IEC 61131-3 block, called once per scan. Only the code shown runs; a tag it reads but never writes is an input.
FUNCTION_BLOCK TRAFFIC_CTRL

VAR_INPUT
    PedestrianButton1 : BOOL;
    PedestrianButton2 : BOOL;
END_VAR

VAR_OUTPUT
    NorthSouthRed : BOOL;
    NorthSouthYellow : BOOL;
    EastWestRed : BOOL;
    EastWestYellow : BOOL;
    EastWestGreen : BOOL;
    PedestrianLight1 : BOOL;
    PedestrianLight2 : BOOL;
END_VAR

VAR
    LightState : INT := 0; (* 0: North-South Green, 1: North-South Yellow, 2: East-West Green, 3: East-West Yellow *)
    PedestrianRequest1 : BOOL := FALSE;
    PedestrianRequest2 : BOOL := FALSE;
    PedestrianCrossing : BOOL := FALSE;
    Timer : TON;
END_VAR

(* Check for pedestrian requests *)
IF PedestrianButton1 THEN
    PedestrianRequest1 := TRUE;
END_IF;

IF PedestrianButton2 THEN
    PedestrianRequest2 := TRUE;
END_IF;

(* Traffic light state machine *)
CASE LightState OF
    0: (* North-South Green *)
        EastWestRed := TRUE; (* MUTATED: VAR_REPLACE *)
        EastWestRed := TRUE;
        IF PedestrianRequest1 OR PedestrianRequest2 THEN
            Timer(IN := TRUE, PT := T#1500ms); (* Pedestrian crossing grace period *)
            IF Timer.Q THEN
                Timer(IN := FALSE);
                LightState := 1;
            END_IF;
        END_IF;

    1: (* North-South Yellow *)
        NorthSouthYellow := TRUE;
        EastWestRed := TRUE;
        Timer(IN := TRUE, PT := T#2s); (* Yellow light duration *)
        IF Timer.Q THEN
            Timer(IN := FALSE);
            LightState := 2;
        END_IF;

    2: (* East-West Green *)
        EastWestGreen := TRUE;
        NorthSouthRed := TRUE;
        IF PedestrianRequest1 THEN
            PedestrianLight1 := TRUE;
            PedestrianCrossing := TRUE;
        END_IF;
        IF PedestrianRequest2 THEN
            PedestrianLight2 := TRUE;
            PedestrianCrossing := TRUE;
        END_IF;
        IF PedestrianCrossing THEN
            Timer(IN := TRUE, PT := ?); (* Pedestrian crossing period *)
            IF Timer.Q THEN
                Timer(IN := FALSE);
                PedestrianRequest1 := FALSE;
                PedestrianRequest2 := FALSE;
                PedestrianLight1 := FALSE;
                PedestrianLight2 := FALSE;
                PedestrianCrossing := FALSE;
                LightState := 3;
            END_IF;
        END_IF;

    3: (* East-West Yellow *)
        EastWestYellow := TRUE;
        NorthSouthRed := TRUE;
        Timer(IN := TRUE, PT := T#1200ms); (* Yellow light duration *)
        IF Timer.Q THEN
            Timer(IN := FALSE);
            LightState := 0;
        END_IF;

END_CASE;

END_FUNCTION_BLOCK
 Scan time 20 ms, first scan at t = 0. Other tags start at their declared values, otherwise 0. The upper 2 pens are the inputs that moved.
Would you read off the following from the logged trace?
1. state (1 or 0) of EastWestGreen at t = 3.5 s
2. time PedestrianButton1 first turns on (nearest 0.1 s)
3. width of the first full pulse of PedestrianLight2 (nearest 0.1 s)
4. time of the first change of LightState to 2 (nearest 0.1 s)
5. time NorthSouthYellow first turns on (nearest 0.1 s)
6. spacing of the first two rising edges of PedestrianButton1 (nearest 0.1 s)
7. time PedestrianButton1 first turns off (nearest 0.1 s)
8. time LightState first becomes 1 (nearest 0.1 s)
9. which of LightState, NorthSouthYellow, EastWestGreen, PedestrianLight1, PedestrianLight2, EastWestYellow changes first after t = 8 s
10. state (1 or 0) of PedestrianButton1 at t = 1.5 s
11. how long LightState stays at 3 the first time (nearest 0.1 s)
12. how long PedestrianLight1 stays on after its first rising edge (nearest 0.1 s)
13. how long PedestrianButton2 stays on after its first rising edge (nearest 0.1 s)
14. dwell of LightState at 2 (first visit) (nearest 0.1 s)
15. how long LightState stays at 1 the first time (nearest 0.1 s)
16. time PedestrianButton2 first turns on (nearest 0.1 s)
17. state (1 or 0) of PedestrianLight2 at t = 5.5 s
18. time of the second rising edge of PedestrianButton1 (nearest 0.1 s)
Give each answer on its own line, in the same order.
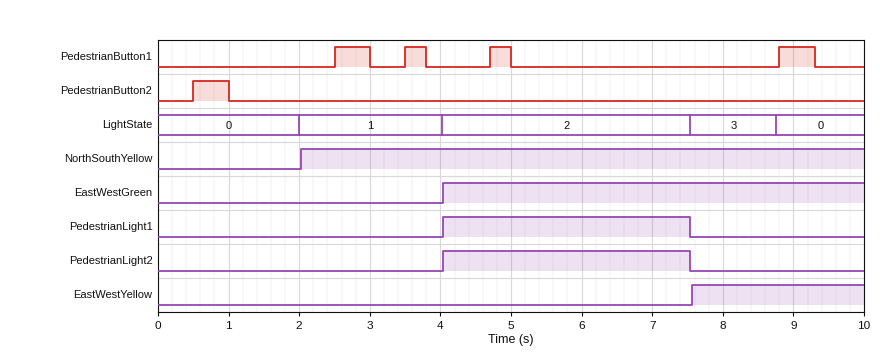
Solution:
0
2.5 s
3.5 s
4.0 s
2.0 s
1.0 s
3.0 s
2.0 s
LightState
0
1.2 s
3.5 s
0.5 s
3.5 s
2.0 s
0.5 s
1
3.5 s
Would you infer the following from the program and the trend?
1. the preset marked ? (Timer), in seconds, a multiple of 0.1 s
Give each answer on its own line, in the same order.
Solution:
3.5 s
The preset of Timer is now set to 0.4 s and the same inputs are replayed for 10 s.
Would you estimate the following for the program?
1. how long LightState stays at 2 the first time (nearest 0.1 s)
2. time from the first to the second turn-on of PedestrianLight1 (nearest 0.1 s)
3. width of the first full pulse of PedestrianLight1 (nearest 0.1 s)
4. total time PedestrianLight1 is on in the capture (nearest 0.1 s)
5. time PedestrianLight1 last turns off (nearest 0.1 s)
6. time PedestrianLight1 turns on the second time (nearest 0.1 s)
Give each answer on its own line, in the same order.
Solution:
0.4 s
5.2 s
0.4 s
0.8 s
9.6 s
9.2 s
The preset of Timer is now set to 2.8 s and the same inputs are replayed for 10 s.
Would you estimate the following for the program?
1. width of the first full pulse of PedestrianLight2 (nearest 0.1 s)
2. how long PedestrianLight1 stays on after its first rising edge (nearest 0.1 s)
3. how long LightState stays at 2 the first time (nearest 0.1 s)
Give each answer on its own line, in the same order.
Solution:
2.8 s
2.8 s
2.8 s
